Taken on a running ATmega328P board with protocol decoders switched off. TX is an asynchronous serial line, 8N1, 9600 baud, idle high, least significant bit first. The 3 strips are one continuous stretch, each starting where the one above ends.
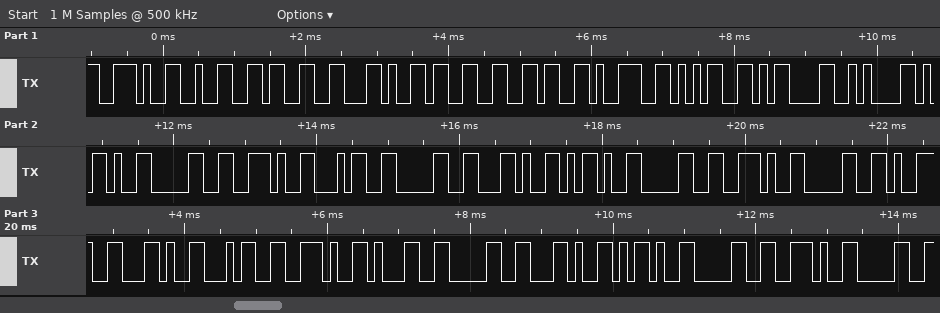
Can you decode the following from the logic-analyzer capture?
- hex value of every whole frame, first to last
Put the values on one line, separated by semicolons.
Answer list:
0x2E 0x32 0x33 0x2C 0x33 0x36 0x39 0x35 0x0D 0x0A 0x2D 0x30 0x2E 0x34 0x30 0x2C 0x2D 0x30 0x2E 0x30 0x39 0x2C 0x34 0x2E 0x31 0x30 0x2C 0x2D 0x30 0x2E 0x30
